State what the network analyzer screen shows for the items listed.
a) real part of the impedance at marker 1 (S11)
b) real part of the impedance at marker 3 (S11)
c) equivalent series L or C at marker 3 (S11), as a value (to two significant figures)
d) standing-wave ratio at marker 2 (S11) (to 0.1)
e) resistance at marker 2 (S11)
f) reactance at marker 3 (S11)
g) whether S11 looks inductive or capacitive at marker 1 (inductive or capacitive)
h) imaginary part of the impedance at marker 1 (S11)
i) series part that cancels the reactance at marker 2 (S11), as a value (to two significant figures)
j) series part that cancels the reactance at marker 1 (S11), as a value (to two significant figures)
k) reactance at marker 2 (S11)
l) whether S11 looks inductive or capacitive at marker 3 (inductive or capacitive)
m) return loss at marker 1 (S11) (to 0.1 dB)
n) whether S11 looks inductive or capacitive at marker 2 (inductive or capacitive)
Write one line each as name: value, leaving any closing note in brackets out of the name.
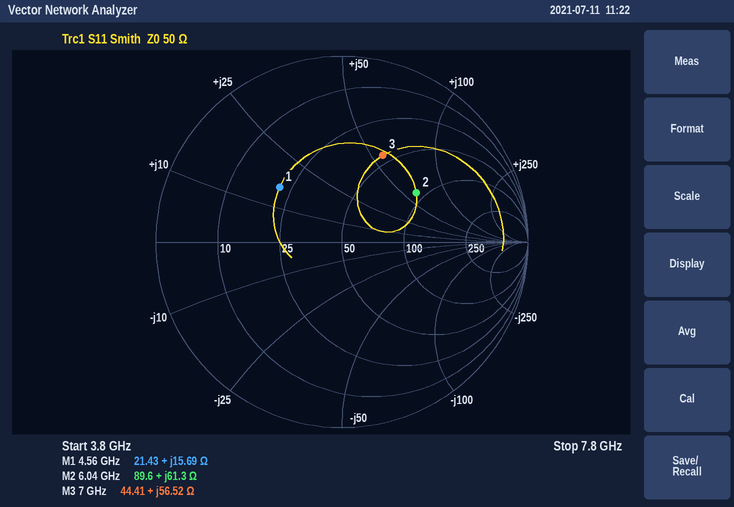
real part of the impedance at marker 1: 21.43 Ω
real part of the impedance at marker 3: 44.41 Ω
equivalent series L or C at marker 3 (S11), as a value: 1.3 nH
standing-wave ratio at marker 2 (S11): 2.8
resistance at marker 2: 89.6 Ω
reactance at marker 3: +56.52 Ω
whether S11 looks inductive or capacitive at marker 1: inductive
imaginary part of the impedance at marker 1: +15.69 Ω
series part that cancels the reactance at marker 2 (S11), as a value: 430 fF
series part that cancels the reactance at marker 1 (S11), as a value: 2.2 pF
reactance at marker 2: +61.3 Ω
whether S11 looks inductive or capacitive at marker 3: inductive
return loss at marker 1 (S11): 7.0 dB
whether S11 looks inductive or capacitive at marker 2: inductive
